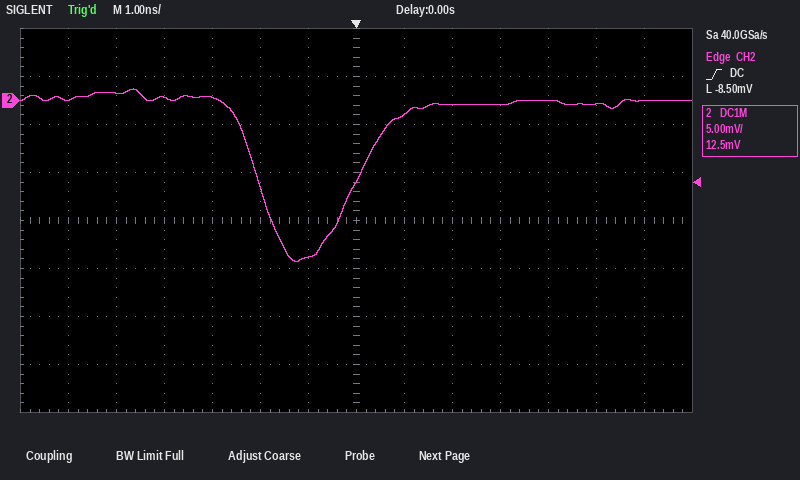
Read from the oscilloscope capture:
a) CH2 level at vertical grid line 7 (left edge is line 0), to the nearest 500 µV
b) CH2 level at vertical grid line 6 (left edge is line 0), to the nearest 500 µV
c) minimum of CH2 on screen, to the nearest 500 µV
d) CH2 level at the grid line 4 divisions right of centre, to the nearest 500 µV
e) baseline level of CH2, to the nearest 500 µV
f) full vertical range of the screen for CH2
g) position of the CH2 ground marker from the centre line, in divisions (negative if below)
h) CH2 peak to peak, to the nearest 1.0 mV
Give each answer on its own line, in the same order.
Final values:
-8.5 mV
-16.5 mV
-17.0 mV
0.0 mV
0.0 mV
40 mV
+2.5 div
18.0 mV
